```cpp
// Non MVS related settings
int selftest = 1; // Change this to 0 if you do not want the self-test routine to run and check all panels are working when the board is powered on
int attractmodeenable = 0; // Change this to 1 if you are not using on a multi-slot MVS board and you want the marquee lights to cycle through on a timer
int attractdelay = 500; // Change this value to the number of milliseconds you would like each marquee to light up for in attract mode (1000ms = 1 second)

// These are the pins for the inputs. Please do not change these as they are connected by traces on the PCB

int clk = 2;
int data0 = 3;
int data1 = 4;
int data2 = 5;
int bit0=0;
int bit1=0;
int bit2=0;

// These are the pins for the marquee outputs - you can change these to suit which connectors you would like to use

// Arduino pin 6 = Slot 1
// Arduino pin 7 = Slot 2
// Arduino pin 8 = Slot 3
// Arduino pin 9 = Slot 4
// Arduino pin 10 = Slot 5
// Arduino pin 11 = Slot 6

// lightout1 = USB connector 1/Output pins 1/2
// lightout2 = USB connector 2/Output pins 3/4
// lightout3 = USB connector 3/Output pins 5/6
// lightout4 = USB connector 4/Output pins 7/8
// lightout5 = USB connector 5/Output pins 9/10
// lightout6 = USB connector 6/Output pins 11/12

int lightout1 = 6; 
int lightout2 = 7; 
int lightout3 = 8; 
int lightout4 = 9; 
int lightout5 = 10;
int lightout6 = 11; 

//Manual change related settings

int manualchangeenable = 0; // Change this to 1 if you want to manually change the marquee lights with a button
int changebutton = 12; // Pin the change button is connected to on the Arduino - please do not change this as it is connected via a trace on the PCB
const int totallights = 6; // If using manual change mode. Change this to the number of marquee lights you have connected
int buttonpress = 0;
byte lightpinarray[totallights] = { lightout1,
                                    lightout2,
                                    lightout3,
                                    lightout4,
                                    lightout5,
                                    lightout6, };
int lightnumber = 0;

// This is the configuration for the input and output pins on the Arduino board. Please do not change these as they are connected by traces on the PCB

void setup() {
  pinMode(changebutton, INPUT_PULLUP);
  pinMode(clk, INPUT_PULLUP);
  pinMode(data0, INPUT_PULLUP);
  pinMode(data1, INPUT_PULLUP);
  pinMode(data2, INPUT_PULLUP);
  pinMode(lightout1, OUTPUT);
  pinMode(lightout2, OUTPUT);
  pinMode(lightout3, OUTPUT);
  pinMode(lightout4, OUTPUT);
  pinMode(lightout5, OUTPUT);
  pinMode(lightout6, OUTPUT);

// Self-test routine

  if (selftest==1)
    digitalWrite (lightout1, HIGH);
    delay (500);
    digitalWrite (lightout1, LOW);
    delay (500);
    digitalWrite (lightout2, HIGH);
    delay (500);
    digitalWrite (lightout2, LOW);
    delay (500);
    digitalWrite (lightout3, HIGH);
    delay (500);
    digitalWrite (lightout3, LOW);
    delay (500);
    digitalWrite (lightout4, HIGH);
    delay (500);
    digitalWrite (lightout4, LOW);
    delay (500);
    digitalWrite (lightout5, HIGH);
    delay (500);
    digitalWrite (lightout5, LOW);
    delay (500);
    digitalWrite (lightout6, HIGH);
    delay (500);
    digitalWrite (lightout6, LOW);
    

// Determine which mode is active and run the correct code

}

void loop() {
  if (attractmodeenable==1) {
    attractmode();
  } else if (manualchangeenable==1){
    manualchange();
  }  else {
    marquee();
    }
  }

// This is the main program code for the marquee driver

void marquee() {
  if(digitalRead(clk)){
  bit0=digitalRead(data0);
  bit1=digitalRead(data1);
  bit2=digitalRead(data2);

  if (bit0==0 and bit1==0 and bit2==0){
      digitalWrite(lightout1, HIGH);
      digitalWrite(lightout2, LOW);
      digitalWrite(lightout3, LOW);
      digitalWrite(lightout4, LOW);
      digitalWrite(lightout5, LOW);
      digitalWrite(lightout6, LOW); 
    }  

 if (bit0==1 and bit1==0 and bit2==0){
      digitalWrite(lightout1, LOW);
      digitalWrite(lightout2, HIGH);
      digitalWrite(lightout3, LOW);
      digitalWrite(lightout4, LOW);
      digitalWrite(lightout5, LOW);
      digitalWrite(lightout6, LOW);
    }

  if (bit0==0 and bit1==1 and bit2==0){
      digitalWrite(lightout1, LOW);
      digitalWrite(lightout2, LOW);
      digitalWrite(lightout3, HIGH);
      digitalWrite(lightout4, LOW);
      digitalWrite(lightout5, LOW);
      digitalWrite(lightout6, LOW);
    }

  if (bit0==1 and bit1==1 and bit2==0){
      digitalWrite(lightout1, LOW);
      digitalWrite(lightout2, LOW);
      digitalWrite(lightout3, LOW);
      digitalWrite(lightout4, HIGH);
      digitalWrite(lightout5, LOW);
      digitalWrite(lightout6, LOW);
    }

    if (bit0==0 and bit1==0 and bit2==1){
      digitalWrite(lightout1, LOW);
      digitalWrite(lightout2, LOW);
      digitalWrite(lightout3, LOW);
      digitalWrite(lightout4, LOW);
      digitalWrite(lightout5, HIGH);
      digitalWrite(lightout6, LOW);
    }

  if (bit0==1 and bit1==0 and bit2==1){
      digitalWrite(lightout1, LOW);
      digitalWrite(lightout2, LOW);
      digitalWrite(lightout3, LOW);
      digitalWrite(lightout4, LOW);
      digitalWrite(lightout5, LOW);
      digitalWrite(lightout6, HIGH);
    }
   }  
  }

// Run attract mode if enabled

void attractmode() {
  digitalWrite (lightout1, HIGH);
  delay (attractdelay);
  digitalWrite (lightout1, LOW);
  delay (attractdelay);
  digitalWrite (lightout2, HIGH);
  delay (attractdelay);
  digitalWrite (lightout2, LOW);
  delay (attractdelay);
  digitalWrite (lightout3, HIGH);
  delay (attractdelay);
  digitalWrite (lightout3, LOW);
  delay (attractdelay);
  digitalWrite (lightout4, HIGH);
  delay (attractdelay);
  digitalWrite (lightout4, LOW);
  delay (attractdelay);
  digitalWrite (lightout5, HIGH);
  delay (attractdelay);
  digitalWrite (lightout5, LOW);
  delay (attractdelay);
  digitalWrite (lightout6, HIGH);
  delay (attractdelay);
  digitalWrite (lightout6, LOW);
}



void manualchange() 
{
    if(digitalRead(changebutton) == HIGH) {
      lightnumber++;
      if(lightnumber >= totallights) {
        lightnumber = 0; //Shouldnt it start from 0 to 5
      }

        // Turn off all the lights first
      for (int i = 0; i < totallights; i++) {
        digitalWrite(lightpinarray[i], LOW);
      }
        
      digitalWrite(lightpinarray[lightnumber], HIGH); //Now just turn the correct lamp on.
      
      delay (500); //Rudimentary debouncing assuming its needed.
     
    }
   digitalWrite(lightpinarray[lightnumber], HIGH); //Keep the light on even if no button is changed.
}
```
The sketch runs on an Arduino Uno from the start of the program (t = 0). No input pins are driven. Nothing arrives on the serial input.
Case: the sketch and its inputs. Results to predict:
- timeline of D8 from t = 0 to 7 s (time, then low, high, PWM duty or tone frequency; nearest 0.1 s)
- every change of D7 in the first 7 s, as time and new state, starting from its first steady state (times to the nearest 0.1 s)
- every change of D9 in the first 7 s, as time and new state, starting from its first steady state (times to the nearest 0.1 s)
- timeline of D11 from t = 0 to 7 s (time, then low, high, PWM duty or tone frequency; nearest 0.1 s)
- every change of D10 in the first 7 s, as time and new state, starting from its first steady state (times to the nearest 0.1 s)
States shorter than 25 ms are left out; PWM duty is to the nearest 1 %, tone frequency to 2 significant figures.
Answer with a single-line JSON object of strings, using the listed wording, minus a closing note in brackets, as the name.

{"timeline of D8 from t = 0 to 7 s": "0 s low; 2 s high; 2.5 s low", "every change of D7 in the first 7 s, as time and new state, starting from its first steady state": "0 s low; 1 s high; 1.5 s low", "every change of D9 in the first 7 s, as time and new state, starting from its first steady state": "0 s low; 3 s high; 3.5 s low", "timeline of D11 from t = 0 to 7 s": "0 s low; 5 s high; 5.5 s low", "every change of D10 in the first 7 s, as time and new state, starting from its first steady state": "0 s low; 4 s high; 4.5 s low"}
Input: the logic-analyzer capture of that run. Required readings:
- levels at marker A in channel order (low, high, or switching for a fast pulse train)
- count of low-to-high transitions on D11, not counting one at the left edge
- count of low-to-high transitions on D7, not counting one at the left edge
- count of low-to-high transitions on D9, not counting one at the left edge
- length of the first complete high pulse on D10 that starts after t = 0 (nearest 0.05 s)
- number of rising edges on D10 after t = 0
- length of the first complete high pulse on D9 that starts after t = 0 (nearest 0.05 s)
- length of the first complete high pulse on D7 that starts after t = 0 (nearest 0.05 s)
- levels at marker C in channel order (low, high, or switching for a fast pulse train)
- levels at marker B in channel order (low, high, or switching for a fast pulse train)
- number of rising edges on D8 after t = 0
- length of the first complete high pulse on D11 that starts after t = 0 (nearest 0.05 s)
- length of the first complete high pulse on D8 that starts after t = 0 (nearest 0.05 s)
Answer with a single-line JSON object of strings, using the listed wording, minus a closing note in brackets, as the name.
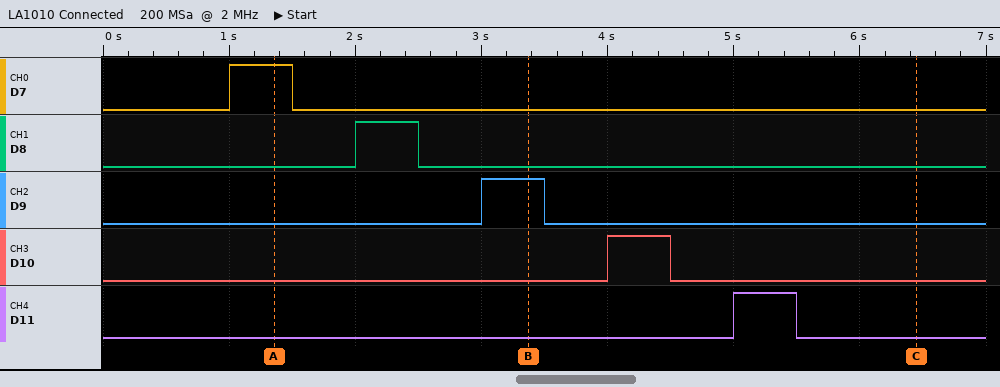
{"levels at marker A in channel order": "D7 high, D8 low, D9 low, D10 low, D11 low", "count of low-to-high transitions on D11, not counting one at the left edge": "1", "count of low-to-high transitions on D7, not counting one at the left edge": "1", "count of low-to-high transitions on D9, not counting one at the left edge": "1", "length of the first complete high pulse on D10 that starts after t = 0": "0.50 s", "number of rising edges on D10 after t = 0": "1", "length of the first complete high pulse on D9 that starts after t = 0": "0.50 s", "length of the first complete high pulse on D7 that starts after t = 0": "0.50 s", "levels at marker C in channel order": "D7 low, D8 low, D9 low, D10 low, D11 low", "levels at marker B in channel order": "D7 low, D8 low, D9 high, D10 low, D11 low", "number of rising edges on D8 after t = 0": "1", "length of the first complete high pulse on D11 that starts after t = 0": "0.50 s", "length of the first complete high pulse on D8 that starts after t = 0": "0.50 s"}
